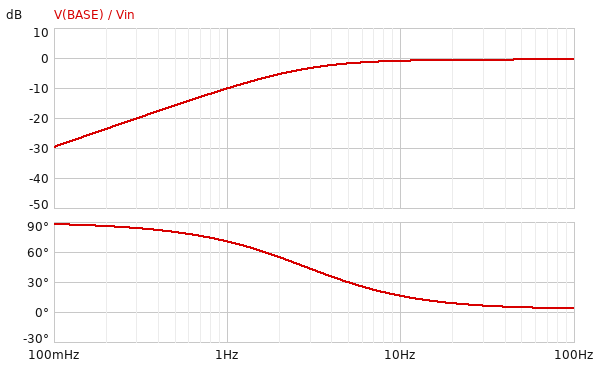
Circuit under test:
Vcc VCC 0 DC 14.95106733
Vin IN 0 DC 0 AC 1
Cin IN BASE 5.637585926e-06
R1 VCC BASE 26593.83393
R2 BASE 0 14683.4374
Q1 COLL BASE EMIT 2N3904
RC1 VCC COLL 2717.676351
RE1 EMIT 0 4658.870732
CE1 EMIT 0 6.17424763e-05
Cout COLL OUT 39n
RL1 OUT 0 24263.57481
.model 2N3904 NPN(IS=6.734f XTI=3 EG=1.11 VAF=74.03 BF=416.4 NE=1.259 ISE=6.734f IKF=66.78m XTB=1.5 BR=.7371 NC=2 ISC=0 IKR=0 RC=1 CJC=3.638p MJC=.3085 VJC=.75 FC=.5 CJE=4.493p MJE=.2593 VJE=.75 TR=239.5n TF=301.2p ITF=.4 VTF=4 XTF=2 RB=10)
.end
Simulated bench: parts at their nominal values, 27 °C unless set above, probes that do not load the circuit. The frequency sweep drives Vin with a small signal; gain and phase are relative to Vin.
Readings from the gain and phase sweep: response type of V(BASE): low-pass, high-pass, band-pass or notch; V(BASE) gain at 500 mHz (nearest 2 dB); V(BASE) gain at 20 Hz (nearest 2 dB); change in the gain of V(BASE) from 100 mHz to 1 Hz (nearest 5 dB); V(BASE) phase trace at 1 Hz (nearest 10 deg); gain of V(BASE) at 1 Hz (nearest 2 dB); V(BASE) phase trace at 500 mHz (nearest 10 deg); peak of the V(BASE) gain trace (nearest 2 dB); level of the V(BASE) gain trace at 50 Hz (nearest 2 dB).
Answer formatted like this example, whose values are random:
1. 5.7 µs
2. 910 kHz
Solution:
1. high-pass
2. -16 dB
3. 0 dB
4. 20 dB
5. 70 deg
6. -10 dB
7. 80 deg
8. 0 dB
9. 0 dB
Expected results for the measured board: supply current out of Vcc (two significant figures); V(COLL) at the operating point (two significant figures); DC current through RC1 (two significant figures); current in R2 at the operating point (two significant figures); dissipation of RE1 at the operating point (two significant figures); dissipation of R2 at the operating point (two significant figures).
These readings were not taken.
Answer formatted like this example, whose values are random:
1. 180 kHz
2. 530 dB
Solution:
1. 1.3 mA
2. 12 V
3. 980 µA
4. 360 µA
5. 4.5 mW
6. 1.9 mW
